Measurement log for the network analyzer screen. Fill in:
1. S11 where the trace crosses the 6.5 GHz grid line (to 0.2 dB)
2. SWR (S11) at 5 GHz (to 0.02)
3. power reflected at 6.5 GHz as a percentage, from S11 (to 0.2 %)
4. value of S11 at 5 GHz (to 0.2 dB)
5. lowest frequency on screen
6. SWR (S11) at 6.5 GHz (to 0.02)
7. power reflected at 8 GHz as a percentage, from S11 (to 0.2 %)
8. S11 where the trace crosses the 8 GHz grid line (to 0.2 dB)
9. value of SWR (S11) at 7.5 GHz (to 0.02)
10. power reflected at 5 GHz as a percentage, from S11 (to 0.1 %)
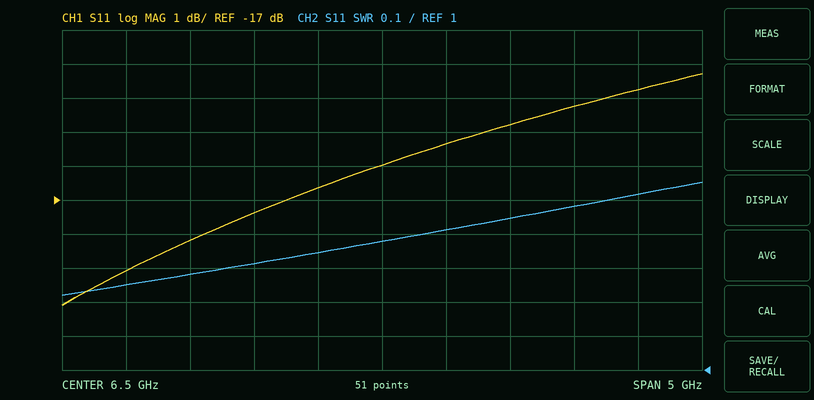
-16.0 dB
1.28
2.6 %
-18.2 dB
4 GHz
1.38
3.8 %
-14.2 dB
1.44
1.5 %
